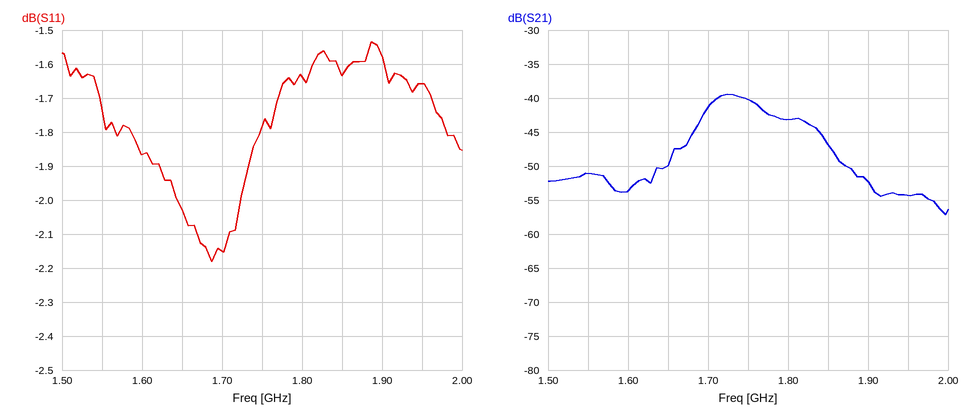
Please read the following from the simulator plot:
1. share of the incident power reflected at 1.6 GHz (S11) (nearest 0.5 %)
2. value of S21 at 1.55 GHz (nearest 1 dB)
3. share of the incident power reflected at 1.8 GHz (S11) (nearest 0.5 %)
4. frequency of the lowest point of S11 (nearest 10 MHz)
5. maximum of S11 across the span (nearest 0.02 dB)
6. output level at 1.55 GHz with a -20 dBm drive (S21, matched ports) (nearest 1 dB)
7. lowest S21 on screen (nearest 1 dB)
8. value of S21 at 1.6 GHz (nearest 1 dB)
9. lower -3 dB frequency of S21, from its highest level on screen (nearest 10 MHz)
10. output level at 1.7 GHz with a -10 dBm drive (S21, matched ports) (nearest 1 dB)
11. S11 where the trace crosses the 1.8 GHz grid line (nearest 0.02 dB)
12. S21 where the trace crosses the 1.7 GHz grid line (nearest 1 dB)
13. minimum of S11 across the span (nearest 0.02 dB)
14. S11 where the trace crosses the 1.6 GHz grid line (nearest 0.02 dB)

65.0 %
-51 dB
68.5 %
1.69 GHz
-1.54 dB
-71 dBm
-57 dB
-54 dB
1.69 GHz
-51 dBm
-1.64 dB
-41 dB
-2.18 dB
-1.86 dB
